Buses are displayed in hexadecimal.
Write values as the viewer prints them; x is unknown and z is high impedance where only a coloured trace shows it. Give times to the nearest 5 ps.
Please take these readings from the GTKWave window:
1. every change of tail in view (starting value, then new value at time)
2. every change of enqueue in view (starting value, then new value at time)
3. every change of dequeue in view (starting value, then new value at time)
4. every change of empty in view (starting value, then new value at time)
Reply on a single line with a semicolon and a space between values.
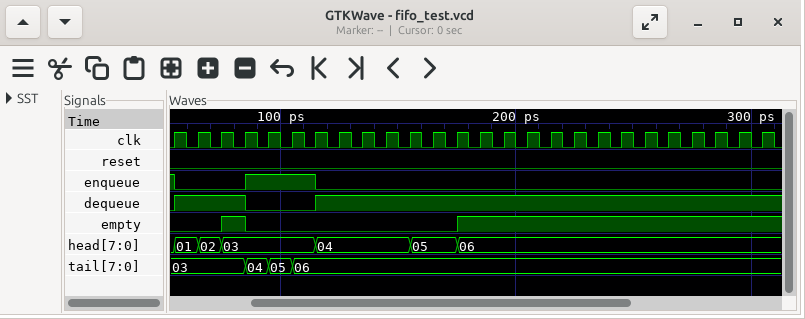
03, 04 at 85 ps, 05 at 95 ps, 06 at 105 ps; 1, 0 at 55 ps, 1 at 85 ps, 0 at 115 ps; 0, 1 at 55 ps, 0 at 85 ps, 1 at 115 ps; 0, 1 at 75 ps, 0 at 85 ps, 1 at 175 ps
